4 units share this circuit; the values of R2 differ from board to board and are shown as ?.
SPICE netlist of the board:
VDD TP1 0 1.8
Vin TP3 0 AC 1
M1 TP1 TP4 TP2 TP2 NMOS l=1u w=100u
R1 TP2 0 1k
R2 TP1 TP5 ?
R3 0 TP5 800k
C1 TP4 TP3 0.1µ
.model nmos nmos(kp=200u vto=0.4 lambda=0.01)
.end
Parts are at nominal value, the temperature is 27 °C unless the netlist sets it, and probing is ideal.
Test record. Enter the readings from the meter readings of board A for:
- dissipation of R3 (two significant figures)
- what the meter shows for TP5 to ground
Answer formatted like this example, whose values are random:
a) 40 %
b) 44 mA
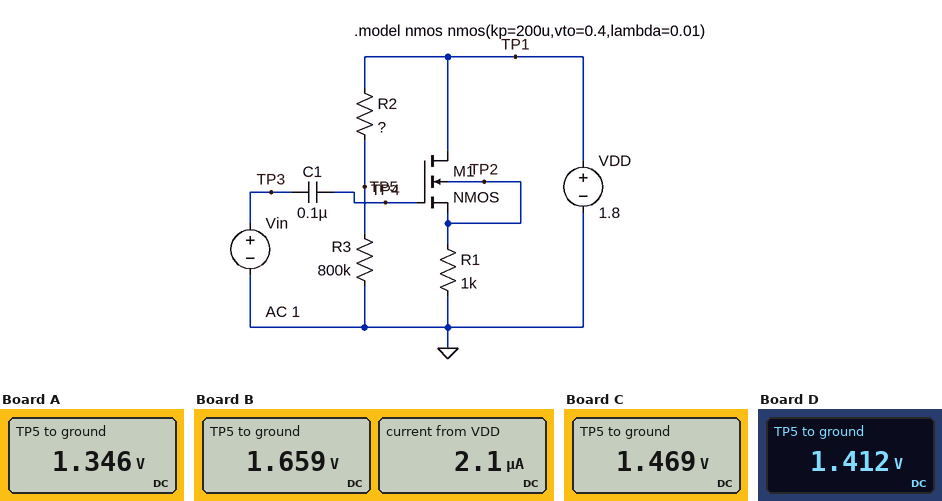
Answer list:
a) 2.3 µW
b) 1.346 V
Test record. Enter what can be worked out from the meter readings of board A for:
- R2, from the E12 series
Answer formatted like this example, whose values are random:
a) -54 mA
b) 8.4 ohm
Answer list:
a) 270 kΩ
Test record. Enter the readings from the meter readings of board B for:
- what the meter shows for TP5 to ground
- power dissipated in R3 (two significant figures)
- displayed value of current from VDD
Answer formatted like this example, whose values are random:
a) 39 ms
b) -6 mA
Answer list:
a) 1.659 V
b) 3.4 µW
c) 2.1 µA
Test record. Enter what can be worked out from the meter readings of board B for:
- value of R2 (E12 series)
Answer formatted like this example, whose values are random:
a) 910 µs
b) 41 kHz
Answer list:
a) 68 kΩ
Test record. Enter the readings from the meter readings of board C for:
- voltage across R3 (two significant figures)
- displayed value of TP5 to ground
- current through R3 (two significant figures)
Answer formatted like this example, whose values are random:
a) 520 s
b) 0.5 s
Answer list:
a) 1.5 V
b) 1.469 V
c) 1.8 µA
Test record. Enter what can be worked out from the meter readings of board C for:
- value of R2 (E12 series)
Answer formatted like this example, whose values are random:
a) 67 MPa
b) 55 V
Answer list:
a) 180 kΩ
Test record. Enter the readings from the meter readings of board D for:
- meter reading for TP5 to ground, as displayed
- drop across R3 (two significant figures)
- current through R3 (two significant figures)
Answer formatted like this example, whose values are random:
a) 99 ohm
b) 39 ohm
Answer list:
a) 1.412 V
b) 1.4 V
c) 1.8 µA
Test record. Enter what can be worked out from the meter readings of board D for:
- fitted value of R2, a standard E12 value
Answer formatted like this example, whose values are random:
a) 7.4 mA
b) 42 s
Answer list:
a) 220 kΩ
